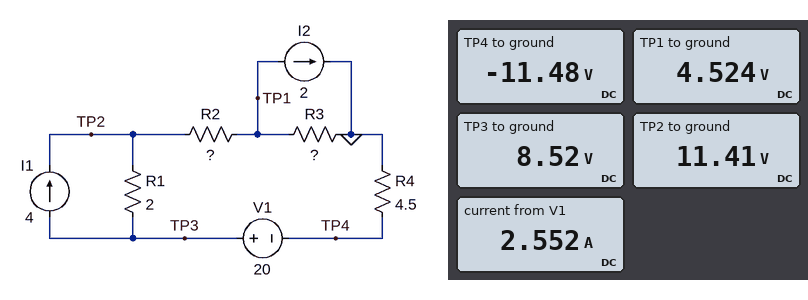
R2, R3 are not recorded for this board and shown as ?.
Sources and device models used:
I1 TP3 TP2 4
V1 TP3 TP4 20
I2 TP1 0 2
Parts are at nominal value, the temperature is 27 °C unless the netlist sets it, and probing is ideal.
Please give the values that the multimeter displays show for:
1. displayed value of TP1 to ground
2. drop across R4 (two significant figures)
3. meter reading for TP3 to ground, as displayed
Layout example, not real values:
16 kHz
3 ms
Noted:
4.524 V
11 V
8.52 V
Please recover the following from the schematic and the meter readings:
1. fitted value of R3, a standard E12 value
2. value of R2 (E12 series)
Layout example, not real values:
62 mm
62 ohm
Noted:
8.2 Ω
2.7 Ω
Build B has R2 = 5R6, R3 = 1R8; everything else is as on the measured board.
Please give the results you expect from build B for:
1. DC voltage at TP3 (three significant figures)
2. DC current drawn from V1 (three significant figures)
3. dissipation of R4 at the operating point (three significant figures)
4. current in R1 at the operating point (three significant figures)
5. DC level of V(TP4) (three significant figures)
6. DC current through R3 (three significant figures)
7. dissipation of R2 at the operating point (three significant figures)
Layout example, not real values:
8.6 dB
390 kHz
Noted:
9.77 V
2.27 A
23.3 W
1.73 A
-10.2 V
273 mA
28.9 W
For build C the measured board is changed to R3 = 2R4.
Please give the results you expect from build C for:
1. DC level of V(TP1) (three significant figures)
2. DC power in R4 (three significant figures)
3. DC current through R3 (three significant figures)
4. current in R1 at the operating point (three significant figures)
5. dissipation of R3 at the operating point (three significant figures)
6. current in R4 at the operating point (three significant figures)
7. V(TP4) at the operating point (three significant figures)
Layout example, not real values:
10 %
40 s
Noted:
1.99 V
36.0 W
828 mA
1.17 A
1.64 W
2.83 A
-12.7 V
